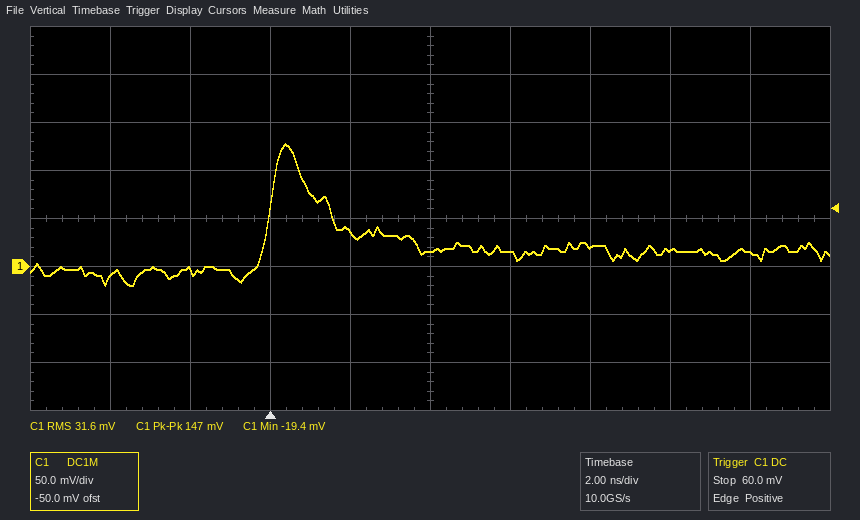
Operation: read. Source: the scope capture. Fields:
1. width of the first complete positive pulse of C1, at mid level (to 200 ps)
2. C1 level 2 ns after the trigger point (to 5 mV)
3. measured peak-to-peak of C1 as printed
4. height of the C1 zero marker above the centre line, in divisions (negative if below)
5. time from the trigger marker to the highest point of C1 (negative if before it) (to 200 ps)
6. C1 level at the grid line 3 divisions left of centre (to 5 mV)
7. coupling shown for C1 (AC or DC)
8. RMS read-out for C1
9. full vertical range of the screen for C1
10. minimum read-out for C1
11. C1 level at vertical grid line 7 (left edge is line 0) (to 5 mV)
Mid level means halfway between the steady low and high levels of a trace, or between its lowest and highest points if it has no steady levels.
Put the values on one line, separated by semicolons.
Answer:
1.6 ns; 35 mV; 147 mV; -1.0 div; +400 ps; -5 mV; DC; 31.6 mV; 400 mV; -19.4 mV; 20 mV
